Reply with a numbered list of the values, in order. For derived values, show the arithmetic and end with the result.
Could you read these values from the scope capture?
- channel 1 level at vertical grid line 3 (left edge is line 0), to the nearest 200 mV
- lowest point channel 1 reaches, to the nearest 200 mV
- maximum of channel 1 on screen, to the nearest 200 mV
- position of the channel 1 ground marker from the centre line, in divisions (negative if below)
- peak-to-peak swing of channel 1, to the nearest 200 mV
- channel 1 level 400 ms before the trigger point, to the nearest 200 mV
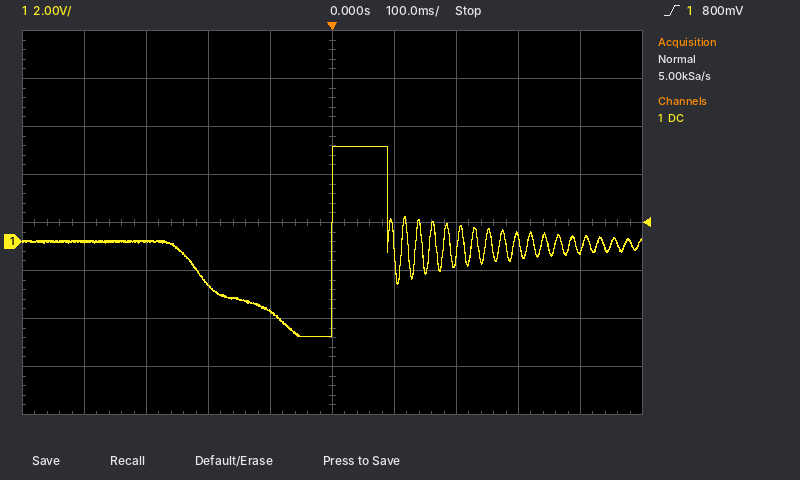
1. -1.8 V
2. -4.0 V
3. 4.0 V
4. -0.4 div
5. 4.0 V − (-4.0 V) = 8.0 V
6. 0.0 V
